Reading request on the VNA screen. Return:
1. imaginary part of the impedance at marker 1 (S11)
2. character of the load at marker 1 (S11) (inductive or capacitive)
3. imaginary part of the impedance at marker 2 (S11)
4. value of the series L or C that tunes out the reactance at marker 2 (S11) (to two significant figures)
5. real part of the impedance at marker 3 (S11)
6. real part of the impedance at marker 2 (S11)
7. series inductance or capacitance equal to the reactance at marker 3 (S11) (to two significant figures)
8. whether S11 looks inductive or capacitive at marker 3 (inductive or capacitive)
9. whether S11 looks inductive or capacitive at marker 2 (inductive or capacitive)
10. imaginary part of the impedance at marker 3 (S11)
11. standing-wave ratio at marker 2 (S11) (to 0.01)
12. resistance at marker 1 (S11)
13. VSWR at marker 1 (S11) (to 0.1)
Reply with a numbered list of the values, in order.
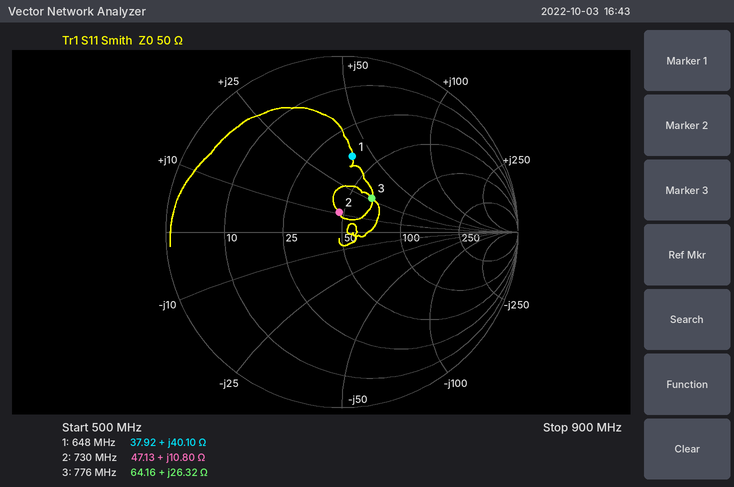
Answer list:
1. +40.10 Ω
2. inductive
3. +10.80 Ω
4. 20 pF
5. 64.16 Ω
6. 47.13 Ω
7. 5.4 nH
8. inductive
9. inductive
10. +26.32 Ω
11. 1.26
12. 37.92 Ω
13. 2.5
